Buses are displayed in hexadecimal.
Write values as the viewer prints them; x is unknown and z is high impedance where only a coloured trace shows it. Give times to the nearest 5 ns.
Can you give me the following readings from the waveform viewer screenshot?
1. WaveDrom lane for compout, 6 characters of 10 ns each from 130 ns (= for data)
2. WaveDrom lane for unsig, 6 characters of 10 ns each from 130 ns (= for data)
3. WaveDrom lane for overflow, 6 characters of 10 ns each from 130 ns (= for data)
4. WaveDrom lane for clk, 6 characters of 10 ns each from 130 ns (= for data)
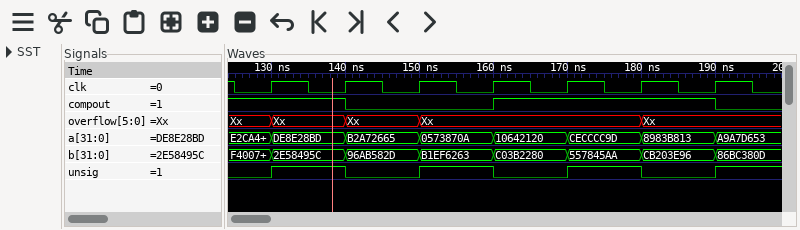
{name: 'compout', wave: '10.1..'}
{name: 'unsig', wave: '101010'}
{name: 'overflow', wave: '===..=', data: 'Xx Xx Xx Xx'}
{name: 'clk', wave: 'p.....'}
